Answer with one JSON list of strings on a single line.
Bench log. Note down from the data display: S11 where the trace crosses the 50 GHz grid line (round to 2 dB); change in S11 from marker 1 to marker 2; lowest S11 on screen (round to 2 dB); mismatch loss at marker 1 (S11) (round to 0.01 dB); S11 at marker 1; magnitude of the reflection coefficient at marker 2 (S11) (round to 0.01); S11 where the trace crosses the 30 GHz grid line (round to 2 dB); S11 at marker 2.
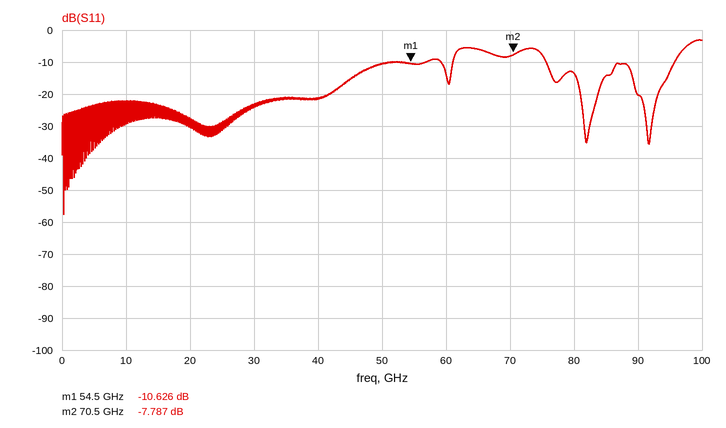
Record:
["-10 dB", "2.839 dB", "-58 dB", "0.39 dB", "-10.626 dB", "0.41", "-24 dB", "-7.787 dB"]
